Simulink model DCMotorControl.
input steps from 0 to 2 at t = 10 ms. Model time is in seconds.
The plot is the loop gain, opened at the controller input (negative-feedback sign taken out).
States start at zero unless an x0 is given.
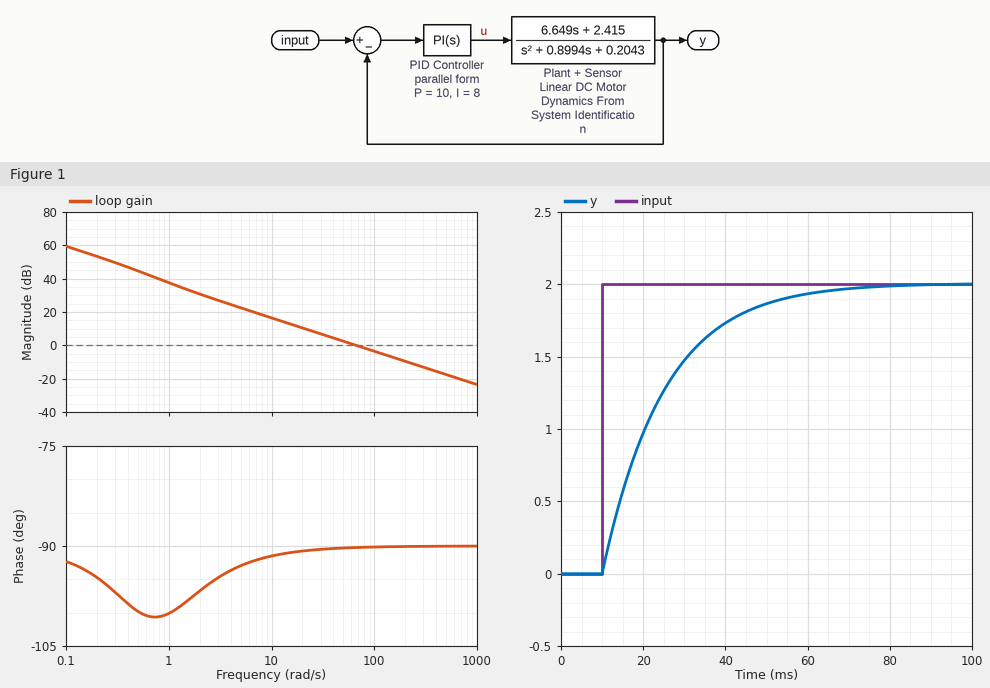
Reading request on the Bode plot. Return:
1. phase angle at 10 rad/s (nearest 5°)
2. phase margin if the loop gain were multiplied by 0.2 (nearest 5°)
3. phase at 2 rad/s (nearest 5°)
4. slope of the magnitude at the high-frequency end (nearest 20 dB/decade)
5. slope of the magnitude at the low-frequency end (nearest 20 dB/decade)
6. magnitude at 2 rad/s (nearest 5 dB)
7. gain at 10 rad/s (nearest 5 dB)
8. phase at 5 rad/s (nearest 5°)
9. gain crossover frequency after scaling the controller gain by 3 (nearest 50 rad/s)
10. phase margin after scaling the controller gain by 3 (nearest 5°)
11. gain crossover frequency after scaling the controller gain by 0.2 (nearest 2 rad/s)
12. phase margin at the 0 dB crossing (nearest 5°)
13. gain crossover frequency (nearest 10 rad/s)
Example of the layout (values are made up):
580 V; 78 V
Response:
-90°; 90°; -95°; -20 dB/decade; -20 dB/decade; 30 dB; 15 dB; -95°; 200 rad/s; 90°; 14 rad/s; 90°; 70 rad/s
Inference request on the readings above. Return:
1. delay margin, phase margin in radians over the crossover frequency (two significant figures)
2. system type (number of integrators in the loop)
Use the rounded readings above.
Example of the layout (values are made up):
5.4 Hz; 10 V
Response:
0.022 s; 1
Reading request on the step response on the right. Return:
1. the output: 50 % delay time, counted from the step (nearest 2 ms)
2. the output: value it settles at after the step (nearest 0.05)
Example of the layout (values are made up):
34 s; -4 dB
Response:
10 ms; 2.00
